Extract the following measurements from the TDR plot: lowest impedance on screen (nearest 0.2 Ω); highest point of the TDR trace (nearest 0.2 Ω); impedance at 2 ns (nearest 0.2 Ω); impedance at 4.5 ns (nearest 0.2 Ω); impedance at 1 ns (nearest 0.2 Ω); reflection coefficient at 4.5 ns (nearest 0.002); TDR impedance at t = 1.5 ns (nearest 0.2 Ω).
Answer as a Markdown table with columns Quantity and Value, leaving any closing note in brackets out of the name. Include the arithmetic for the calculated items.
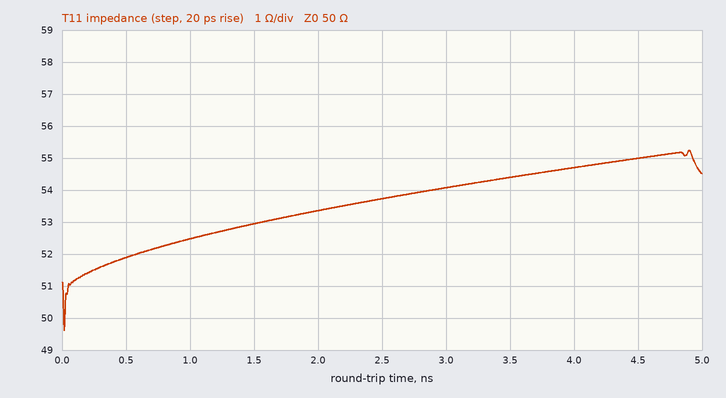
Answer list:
| Quantity | Value |
|---|---|
| lowest impedance on screen | 49.6 Ω |
| highest point of the TDR trace | 55.2 Ω |
| impedance at 2 ns | 53.4 Ω |
| impedance at 4.5 ns | 55.0 Ω |
| impedance at 1 ns | 52.4 Ω |
| reflection coefficient at 4.5 ns | (55 − 50)/(55 + 50) ≈ +0.048 |
| TDR impedance at t = 1.5 ns | 53.0 Ω |
